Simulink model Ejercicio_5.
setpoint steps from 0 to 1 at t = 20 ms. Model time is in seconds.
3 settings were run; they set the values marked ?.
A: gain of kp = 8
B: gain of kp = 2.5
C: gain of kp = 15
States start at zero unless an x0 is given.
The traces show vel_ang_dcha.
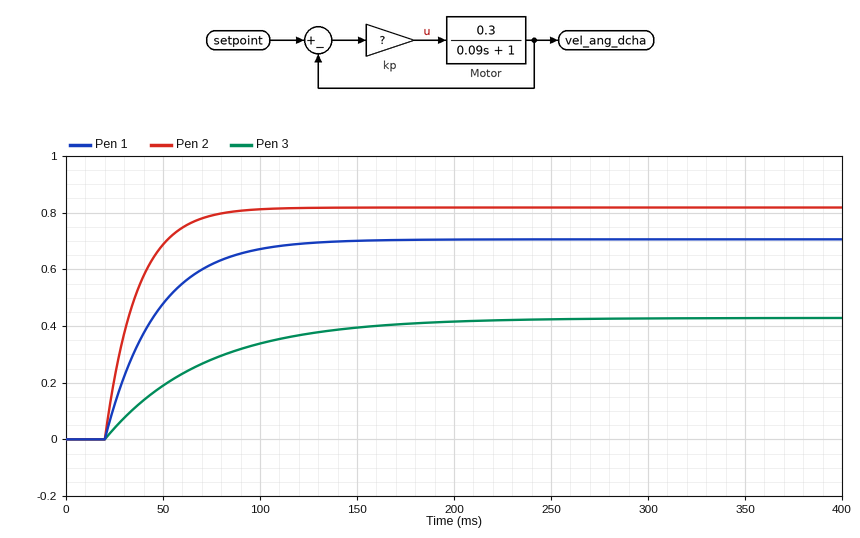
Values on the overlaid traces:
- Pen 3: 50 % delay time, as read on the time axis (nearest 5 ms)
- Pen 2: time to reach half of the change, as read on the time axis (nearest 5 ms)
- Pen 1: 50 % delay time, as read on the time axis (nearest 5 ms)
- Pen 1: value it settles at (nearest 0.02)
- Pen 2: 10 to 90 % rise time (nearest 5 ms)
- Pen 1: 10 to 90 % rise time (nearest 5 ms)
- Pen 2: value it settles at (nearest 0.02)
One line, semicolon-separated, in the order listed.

55 ms; 30 ms; 40 ms; 0.70; 35 ms; 60 ms; 0.82
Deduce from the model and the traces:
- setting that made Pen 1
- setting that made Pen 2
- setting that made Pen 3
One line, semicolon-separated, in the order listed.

A; C; B
